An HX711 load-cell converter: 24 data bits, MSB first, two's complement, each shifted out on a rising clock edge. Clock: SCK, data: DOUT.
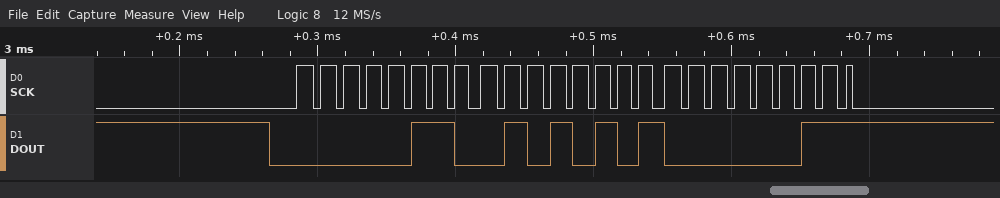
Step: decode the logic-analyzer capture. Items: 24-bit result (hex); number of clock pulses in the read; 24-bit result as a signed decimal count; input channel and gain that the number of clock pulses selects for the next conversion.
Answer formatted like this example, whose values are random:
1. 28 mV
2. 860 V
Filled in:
1. 0x065503
2. 25
3. 414979
4. channel A, gain 128
